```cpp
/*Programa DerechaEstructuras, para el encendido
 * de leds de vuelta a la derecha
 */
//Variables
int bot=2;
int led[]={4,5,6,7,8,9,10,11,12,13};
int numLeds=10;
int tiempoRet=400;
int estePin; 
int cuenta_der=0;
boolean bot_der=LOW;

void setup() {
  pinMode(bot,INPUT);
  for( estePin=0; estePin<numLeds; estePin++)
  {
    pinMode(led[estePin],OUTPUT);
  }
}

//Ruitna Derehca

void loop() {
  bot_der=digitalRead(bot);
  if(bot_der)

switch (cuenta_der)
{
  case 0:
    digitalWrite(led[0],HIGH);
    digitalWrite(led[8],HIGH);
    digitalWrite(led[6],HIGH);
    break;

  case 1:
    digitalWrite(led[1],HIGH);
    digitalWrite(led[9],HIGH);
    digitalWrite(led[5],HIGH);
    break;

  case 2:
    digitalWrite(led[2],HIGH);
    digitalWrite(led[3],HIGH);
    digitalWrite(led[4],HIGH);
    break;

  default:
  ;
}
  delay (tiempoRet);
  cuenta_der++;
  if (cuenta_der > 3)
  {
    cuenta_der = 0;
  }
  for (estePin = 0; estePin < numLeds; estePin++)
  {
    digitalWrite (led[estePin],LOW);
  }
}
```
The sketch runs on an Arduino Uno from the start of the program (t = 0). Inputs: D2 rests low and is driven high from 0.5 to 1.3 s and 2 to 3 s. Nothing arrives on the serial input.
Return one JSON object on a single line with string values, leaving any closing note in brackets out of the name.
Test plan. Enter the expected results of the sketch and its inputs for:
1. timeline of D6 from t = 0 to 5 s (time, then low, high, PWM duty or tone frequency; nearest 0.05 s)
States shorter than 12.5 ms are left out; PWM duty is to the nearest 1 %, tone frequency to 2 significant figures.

{"timeline of D6 from t = 0 to 5 s": "0 s low; 0.8 s high; 1.2 s low; 2.4 s high; 2.8 s low"}
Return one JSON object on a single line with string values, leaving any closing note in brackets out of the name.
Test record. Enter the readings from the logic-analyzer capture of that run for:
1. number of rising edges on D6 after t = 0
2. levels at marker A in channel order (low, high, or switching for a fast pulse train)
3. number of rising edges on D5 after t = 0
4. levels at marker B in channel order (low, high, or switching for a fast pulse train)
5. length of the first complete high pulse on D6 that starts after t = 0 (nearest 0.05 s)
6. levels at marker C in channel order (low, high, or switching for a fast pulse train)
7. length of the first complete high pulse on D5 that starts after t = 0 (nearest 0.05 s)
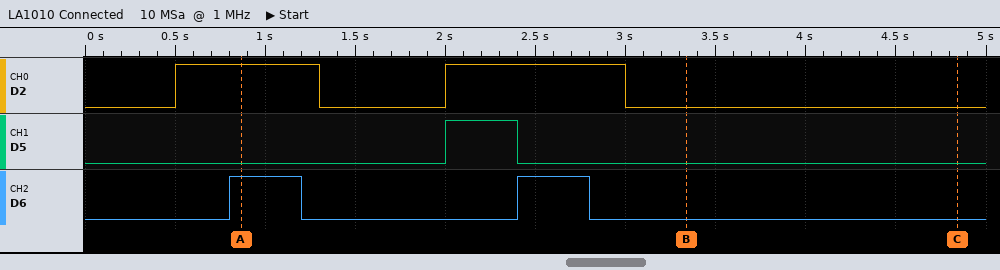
{"number of rising edges on D6 after t = 0": "2", "levels at marker A in channel order": "D2 high, D5 low, D6 high", "number of rising edges on D5 after t = 0": "1", "levels at marker B in channel order": "D2 low, D5 low, D6 low", "length of the first complete high pulse on D6 that starts after t = 0": "0.40 s", "levels at marker C in channel order": "D2 low, D5 low, D6 low", "length of the first complete high pulse on D5 that starts after t = 0": "0.40 s"}
